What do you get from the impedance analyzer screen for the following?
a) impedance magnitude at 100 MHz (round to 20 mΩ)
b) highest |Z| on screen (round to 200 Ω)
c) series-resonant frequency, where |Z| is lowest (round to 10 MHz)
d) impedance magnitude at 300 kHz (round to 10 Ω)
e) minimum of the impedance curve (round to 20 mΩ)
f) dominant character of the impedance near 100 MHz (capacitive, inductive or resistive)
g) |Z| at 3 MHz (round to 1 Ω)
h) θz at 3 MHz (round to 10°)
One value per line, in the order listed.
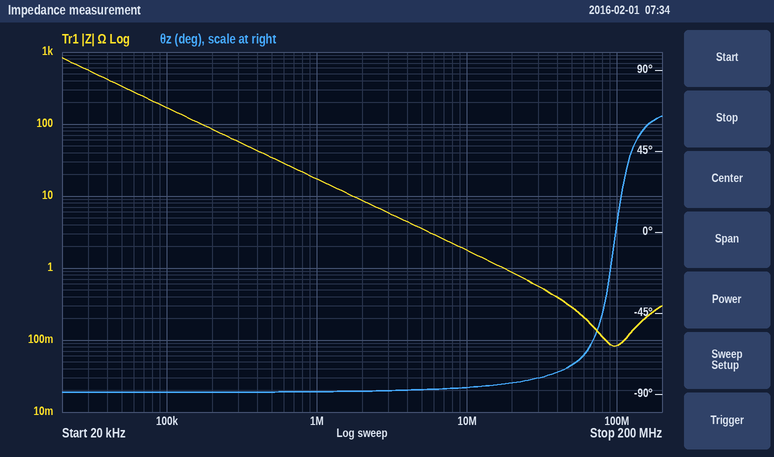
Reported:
80 mΩ
800 Ω
100 MHz
60 Ω
80 mΩ
resistive
6 Ω
-90°
